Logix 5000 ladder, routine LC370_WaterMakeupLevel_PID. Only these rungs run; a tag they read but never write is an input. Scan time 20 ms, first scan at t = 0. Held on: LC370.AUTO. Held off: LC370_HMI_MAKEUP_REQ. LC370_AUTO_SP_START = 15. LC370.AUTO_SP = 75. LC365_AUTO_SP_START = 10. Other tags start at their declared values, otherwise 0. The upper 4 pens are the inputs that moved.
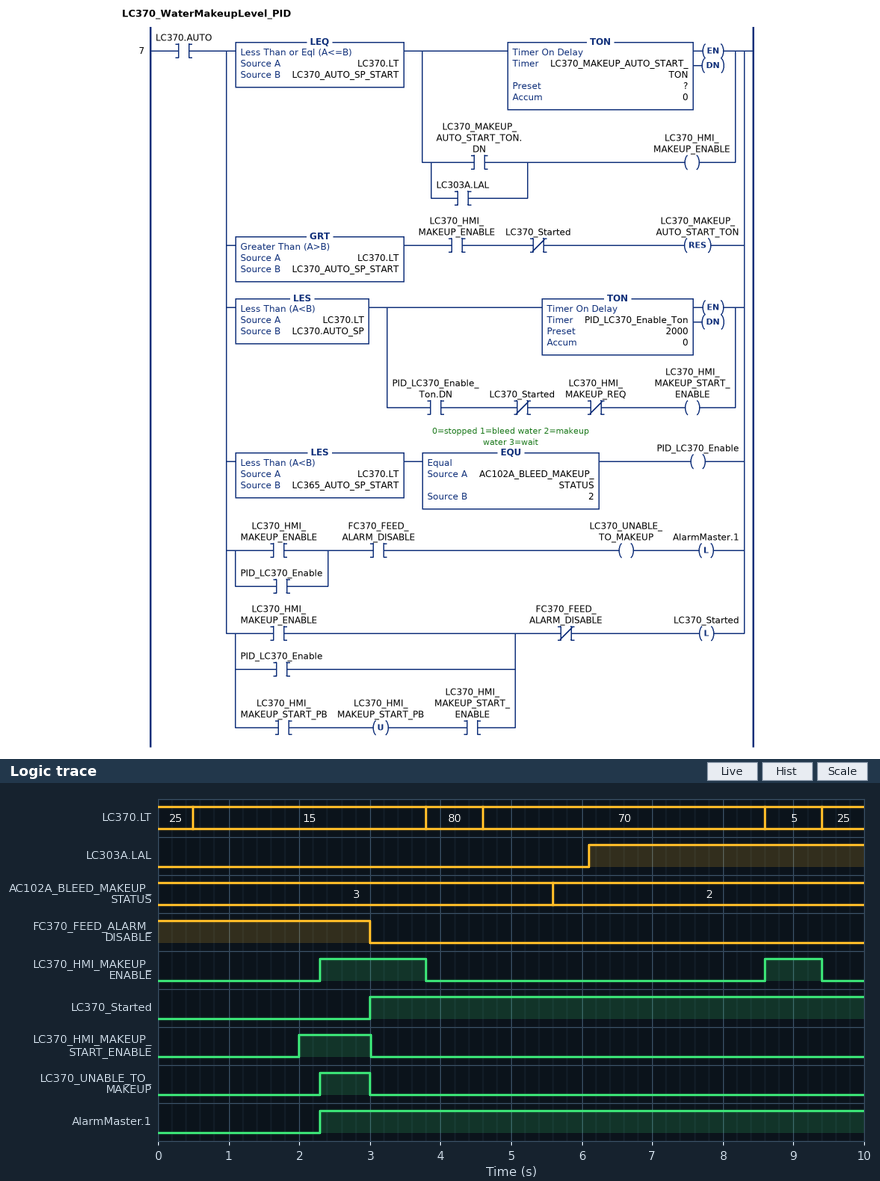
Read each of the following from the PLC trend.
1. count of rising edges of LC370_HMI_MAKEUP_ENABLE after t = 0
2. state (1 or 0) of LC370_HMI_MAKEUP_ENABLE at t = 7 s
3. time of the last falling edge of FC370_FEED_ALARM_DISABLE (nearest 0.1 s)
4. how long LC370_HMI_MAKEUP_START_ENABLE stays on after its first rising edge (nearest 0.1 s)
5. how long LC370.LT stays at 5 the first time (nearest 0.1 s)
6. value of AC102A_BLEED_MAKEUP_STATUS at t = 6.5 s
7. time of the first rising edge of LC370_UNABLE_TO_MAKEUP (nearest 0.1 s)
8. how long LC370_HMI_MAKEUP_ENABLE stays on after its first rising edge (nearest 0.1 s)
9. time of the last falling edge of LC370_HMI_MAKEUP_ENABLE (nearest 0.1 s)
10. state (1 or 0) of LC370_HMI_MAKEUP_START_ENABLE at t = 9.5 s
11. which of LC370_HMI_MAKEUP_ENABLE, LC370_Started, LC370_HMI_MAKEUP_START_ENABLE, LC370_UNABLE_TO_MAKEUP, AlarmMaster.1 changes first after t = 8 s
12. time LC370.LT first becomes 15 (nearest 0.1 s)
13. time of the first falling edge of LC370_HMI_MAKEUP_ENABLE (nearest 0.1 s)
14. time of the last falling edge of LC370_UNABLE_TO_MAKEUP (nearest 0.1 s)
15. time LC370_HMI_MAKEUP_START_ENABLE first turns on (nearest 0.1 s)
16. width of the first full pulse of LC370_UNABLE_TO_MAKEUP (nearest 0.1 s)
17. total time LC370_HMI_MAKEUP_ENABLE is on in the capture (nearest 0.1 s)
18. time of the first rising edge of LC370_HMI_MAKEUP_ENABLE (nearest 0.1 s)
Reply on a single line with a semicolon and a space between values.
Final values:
2; 0; 3.0 s; 1.0 s; 0.8 s; 2; 2.3 s; 1.5 s; 9.4 s; 0; LC370_HMI_MAKEUP_ENABLE; 0.5 s; 3.8 s; 3.0 s; 2.0 s; 0.7 s; 2.3 s; 2.3 s
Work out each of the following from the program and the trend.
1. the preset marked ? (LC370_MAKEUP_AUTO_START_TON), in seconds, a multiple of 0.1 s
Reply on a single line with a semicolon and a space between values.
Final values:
1.8 s
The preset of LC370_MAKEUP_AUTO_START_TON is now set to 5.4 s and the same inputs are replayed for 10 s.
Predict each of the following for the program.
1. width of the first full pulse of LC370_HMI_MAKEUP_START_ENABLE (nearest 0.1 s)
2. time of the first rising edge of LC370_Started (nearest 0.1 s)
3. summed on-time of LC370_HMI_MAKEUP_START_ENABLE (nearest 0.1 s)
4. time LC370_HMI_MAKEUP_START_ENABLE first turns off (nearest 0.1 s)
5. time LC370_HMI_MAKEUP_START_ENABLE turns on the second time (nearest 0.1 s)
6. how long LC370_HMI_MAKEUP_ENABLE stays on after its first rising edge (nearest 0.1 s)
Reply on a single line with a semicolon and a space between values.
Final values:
1.8 s; 8.6 s; 3.8 s; 3.8 s; 6.6 s; 0.8 s
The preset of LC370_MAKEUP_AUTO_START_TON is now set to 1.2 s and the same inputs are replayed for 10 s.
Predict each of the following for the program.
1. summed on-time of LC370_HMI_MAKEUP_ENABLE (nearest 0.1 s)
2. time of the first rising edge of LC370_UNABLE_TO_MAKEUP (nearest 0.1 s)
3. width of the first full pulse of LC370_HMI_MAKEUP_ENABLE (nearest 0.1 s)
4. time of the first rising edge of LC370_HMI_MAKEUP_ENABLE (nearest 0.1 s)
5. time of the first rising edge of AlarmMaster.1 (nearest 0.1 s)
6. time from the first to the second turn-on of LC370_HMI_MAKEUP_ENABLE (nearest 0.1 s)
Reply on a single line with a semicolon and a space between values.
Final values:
2.9 s; 1.7 s; 2.1 s; 1.7 s; 1.7 s; 6.9 s
